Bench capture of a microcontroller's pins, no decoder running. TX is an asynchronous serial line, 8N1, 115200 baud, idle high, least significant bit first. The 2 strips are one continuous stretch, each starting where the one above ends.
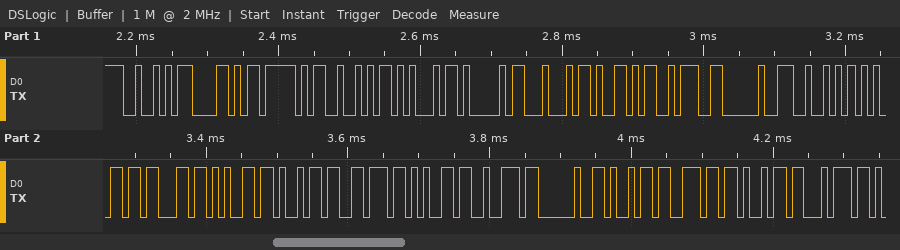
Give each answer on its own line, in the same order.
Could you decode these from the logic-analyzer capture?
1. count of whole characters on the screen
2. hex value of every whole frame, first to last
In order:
23
52 58 5F 52 45 41 44 59 3A 20 52 65 63 65 69 76 65 72 20 69 6E 69 74
